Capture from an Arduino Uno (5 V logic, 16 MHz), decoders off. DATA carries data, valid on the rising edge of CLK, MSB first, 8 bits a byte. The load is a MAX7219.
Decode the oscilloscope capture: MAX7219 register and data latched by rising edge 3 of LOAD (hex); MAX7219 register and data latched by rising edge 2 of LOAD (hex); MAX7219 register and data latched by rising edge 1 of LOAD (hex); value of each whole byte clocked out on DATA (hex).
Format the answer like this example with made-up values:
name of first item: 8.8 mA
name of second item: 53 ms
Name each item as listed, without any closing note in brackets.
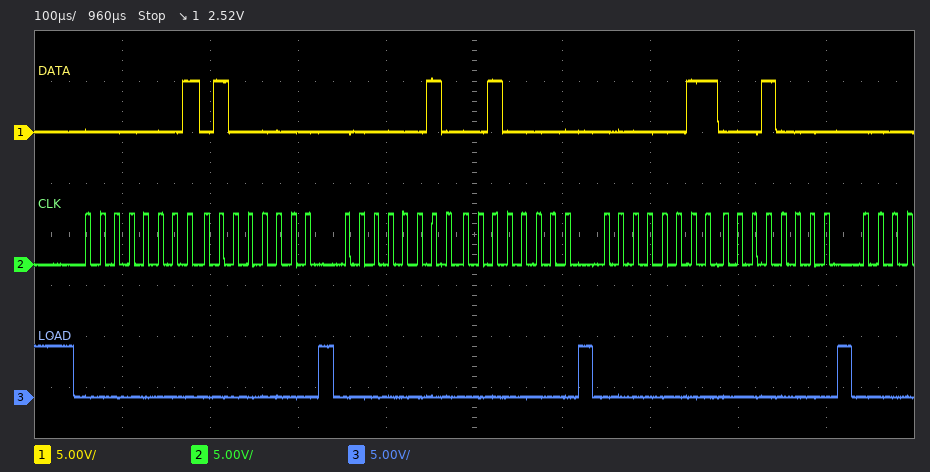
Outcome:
MAX7219 register and data latched by rising edge 3 of LOAD: register 0x3, data 0x10
MAX7219 register and data latched by rising edge 2 of LOAD: register 0x2, data 0x20
MAX7219 register and data latched by rising edge 1 of LOAD: register 0x1, data 0x40
value of each whole byte clocked out on DATA: 0x01 0x40 0x02 0x20 0x03 0x10
